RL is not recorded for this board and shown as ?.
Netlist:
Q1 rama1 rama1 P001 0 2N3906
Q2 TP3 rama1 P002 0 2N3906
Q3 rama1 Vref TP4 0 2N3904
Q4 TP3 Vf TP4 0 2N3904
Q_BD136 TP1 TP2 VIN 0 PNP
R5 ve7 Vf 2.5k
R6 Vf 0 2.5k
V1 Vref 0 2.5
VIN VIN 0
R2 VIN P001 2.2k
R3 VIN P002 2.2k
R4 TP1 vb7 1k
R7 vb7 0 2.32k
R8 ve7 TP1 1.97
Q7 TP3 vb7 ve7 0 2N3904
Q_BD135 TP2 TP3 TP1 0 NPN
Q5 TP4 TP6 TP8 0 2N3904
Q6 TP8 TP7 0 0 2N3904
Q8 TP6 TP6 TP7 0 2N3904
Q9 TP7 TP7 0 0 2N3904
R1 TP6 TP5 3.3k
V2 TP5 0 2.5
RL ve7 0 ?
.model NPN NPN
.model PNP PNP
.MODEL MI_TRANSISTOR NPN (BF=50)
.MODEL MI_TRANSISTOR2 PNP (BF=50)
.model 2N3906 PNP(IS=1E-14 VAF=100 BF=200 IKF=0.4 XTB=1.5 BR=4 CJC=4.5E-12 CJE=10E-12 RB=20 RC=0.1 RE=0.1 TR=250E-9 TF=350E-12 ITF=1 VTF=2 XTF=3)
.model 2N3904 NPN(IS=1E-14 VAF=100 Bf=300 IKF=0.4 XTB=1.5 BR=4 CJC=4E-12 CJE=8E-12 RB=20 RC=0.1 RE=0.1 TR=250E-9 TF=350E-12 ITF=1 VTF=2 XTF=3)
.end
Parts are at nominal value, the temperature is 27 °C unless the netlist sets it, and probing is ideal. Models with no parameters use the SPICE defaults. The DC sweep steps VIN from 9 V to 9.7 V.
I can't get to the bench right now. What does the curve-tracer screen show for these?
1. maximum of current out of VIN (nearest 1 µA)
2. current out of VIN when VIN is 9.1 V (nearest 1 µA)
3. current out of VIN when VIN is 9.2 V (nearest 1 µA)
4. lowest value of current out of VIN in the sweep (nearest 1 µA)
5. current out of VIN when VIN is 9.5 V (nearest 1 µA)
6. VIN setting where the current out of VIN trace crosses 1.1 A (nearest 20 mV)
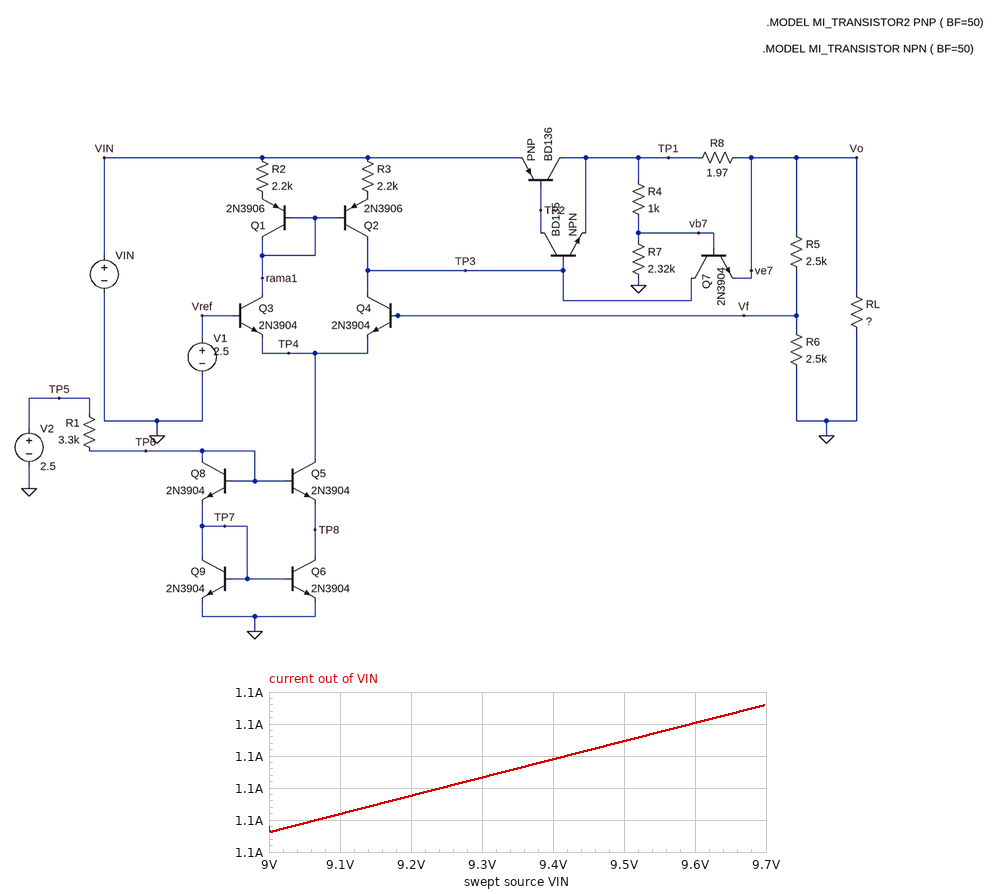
1.102303 A
1.102286 A
1.102289 A
1.102283 A
1.102297 A
9.24 V
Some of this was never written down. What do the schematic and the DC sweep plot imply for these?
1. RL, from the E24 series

2.7 Ω
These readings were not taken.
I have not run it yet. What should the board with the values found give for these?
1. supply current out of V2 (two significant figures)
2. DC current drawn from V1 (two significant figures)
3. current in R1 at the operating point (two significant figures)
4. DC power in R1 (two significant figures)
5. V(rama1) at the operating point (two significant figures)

380 µA
370 µA
380 µA
470 µW
1.8 V
